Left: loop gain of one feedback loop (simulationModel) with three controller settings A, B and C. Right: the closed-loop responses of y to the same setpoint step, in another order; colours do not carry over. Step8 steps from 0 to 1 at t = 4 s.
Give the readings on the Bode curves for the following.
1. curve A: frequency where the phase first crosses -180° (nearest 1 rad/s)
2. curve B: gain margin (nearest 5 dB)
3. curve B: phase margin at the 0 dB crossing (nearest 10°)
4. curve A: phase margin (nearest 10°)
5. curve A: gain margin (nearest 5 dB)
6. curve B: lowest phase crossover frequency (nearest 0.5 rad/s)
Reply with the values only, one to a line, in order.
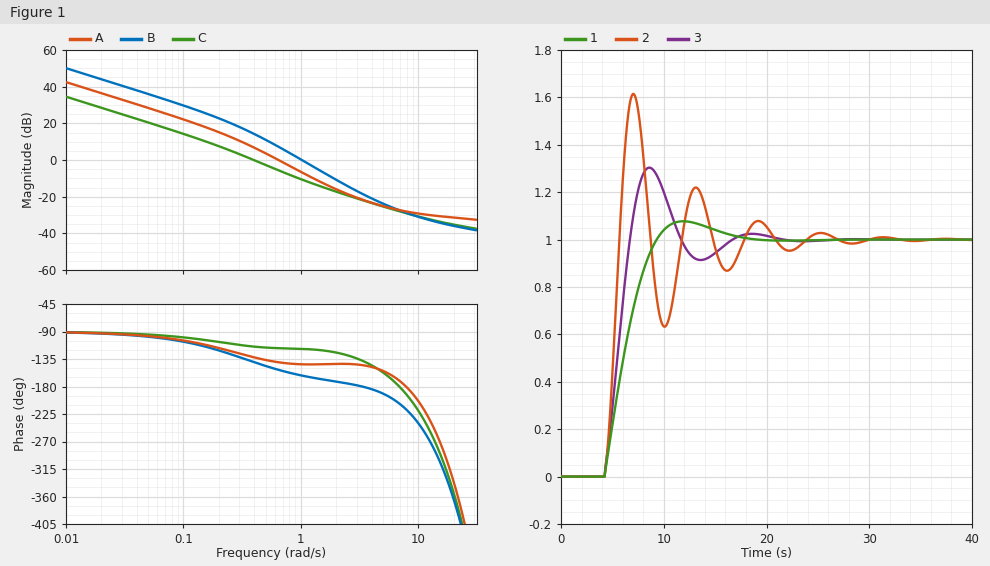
8 rad/s
20 dB
20°
40°
30 dB
3.5 rad/s
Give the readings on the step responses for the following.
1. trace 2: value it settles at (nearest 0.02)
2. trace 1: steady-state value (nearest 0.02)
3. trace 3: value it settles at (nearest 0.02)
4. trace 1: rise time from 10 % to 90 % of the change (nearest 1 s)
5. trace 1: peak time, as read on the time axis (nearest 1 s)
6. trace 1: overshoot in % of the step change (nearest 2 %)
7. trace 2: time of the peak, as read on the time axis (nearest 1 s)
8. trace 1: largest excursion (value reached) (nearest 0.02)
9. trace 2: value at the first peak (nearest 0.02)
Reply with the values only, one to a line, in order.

1.00
1.00
1.00
4 s
12 s
8 %
7 s
1.08
1.62
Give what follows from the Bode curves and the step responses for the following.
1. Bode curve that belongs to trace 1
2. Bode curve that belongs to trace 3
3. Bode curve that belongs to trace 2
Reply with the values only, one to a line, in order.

C
A
B
